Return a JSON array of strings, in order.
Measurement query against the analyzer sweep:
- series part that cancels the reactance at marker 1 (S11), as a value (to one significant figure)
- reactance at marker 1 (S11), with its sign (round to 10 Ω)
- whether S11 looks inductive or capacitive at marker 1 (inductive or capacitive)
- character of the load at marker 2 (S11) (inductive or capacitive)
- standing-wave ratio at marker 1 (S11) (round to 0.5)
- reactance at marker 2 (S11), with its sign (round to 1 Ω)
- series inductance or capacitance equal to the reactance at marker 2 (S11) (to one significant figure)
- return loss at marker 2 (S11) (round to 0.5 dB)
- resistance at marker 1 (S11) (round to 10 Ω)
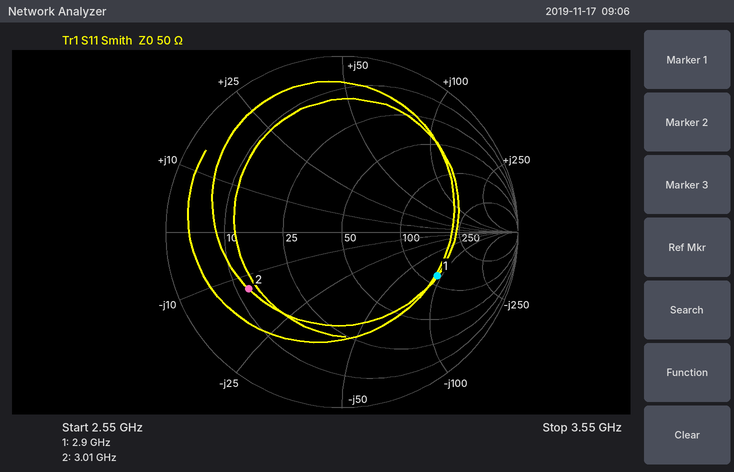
["5 nH", "-90 Ω", "capacitive", "capacitive", "4.0", "-13 Ω", "4 pF", "4.0 dB", "120 Ω"]
